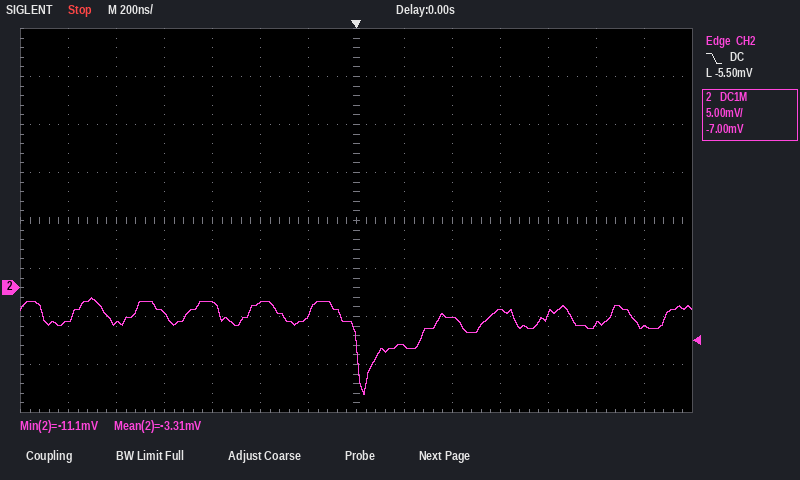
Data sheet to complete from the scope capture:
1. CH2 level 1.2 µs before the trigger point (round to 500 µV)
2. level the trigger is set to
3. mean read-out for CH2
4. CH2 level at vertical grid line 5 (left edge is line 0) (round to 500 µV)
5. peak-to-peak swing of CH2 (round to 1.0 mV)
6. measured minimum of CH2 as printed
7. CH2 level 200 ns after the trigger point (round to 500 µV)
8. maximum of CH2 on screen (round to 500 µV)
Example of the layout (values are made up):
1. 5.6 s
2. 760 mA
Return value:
1. -3.5 mV
2. -5.50 mV
3. -3.31 mV
4. -1.5 mV
5. 10.0 mV
6. -11.1 mV
7. -6.0 mV
8. -1.0 mV
